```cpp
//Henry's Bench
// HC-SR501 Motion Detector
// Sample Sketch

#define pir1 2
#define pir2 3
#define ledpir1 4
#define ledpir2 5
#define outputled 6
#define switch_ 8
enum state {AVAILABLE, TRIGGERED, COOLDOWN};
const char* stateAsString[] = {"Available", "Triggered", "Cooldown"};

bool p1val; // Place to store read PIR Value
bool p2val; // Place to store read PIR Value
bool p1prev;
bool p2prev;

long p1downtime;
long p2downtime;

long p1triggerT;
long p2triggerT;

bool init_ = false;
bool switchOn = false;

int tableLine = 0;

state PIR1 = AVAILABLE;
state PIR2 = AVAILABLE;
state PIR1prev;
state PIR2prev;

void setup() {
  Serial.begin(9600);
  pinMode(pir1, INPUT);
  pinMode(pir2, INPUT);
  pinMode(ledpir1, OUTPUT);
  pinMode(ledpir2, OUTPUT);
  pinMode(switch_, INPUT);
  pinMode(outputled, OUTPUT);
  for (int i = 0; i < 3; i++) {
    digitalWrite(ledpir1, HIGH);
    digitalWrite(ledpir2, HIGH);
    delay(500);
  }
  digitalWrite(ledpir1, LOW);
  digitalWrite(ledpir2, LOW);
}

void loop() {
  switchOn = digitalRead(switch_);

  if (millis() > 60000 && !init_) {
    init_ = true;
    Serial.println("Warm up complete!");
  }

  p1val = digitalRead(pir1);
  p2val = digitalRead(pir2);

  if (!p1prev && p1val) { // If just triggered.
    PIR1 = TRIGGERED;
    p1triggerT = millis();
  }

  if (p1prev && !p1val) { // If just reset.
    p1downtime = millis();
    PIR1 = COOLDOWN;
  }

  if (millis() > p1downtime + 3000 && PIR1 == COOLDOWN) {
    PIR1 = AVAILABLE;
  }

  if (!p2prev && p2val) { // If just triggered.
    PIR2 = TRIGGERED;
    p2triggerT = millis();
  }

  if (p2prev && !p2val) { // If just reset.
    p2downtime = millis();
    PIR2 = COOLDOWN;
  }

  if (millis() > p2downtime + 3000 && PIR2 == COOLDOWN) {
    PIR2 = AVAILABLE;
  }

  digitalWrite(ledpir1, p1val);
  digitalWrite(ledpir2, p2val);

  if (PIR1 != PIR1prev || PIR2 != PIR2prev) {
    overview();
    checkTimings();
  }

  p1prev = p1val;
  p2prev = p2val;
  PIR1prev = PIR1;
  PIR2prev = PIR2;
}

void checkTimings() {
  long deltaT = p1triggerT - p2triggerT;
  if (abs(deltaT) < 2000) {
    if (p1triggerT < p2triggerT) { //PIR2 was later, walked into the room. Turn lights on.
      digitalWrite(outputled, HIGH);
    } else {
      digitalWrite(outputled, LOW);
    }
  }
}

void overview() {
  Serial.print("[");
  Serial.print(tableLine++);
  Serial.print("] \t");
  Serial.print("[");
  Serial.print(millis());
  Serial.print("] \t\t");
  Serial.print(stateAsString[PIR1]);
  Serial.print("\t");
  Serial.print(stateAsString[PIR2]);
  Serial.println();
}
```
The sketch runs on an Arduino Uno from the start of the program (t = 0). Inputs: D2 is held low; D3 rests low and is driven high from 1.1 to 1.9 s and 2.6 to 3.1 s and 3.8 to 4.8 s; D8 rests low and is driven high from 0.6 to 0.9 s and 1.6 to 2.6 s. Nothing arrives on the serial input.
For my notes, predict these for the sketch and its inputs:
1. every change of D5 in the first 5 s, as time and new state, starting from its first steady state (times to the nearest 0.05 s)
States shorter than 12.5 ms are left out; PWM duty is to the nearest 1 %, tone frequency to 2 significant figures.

0 s high; 1.9 s low; 2.6 s high; 3.1 s low; 3.8 s high; 4.8 s low
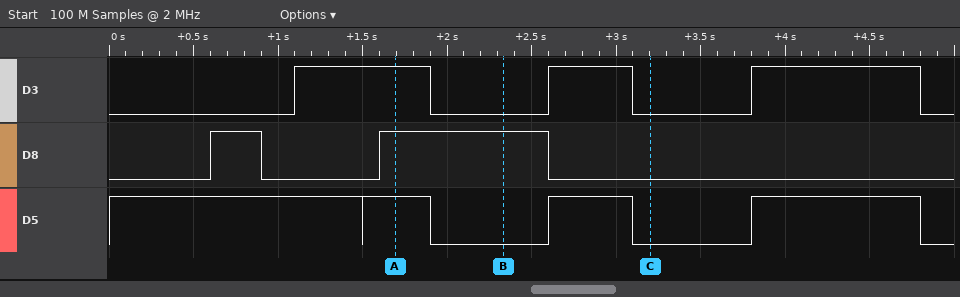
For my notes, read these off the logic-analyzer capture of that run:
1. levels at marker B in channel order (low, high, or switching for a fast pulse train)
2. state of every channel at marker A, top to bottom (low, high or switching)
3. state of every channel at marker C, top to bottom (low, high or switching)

D3 low, D8 high, D5 low
D3 high, D8 high, D5 high
D3 low, D8 low, D5 low
